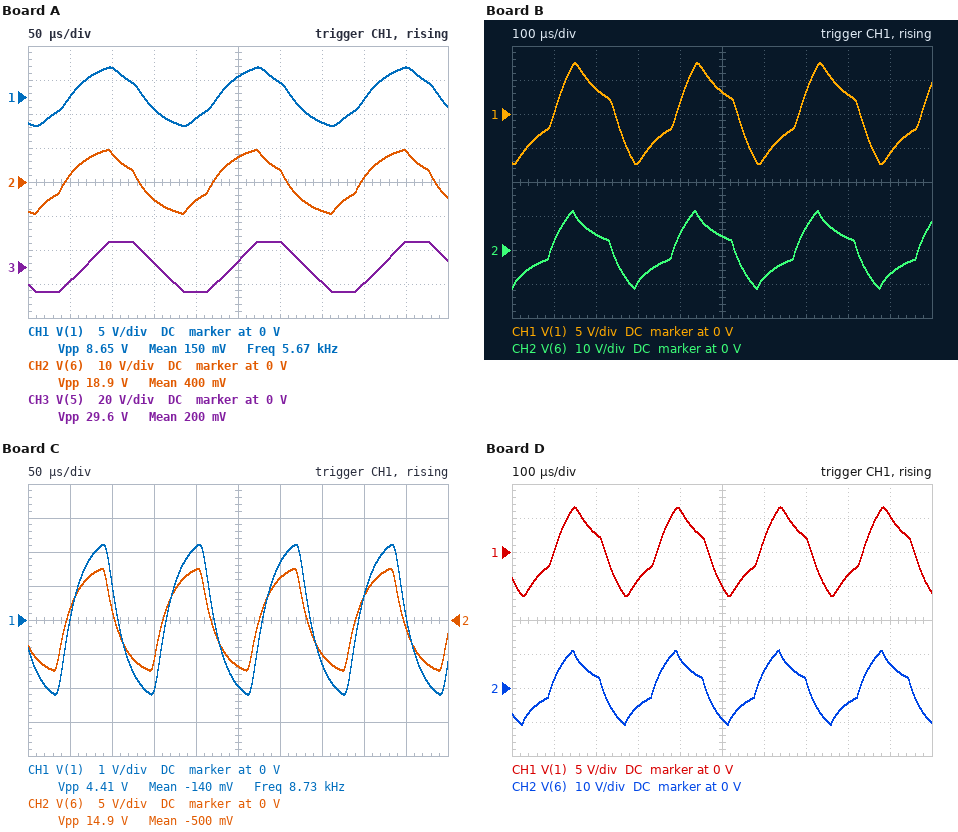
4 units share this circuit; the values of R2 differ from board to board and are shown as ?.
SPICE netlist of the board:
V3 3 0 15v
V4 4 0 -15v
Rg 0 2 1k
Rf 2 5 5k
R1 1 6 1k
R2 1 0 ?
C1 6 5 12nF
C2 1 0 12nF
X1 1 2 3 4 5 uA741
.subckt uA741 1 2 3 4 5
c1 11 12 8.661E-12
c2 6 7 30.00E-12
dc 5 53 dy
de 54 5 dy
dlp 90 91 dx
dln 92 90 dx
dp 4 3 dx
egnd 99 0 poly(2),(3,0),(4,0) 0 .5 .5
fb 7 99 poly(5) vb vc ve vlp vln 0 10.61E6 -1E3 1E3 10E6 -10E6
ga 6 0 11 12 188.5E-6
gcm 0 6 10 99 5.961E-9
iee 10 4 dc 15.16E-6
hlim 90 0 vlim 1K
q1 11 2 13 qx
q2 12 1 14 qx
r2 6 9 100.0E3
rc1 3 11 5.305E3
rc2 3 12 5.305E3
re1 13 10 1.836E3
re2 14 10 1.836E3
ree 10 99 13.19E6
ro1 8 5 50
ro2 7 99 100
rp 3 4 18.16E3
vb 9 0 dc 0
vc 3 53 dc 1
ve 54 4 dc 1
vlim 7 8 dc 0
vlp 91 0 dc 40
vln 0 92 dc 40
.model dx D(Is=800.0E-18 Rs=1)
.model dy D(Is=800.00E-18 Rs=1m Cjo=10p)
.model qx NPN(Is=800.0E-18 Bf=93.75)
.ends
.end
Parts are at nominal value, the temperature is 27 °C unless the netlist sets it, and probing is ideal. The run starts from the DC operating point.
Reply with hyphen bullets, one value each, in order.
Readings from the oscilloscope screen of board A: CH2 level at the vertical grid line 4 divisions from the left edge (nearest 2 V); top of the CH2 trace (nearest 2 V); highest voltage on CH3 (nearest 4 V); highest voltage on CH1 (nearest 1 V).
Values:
- -6 V
- 10 V
- 16 V
- 4 V
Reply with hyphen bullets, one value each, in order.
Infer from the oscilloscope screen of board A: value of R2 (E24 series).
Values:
- 910 Ω
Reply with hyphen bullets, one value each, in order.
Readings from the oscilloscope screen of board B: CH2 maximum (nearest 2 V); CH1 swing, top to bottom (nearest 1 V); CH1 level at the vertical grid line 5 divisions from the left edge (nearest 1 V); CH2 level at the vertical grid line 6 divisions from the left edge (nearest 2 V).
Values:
- 12 V
- 15 V
- 3 V
- -8 V
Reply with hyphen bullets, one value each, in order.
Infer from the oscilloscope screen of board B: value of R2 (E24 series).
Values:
- 2.4 kΩ
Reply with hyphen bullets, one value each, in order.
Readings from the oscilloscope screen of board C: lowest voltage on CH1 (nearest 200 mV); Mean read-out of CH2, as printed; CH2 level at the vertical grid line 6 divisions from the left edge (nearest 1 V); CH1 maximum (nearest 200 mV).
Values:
- -2.2 V
- -500 mV
- 6 V
- 2.2 V
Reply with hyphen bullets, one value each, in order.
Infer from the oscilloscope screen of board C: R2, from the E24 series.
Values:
- 430 Ω
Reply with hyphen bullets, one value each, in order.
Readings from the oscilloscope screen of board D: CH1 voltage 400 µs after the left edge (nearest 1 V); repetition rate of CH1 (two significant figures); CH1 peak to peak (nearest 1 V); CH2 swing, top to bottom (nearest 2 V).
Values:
- 6 V
- 4.1 kHz
- 13 V
- 22 V
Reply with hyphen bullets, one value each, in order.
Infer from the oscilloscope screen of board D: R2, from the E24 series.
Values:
- 1.8 kΩ
